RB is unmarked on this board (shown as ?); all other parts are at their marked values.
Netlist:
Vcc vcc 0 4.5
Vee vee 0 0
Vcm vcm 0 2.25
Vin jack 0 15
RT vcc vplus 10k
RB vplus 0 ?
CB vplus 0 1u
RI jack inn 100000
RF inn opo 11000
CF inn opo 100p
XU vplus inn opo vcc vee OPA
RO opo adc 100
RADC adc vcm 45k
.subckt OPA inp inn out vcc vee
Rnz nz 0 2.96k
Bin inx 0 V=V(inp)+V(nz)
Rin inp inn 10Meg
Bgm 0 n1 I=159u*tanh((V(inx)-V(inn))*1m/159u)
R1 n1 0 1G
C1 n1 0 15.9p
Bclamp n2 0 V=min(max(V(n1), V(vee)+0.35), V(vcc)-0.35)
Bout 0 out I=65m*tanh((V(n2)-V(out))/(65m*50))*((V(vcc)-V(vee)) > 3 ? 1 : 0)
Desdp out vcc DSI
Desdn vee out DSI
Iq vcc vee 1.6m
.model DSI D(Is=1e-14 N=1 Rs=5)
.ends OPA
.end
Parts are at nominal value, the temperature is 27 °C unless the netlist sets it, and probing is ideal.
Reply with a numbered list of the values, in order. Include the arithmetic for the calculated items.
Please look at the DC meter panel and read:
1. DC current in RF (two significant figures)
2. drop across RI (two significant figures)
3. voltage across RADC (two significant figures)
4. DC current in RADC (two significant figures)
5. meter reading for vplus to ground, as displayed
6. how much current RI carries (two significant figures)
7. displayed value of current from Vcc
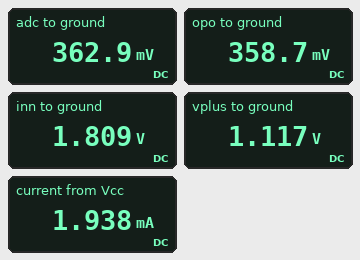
1. (1.809 V - 358.7 mV) / 11 kΩ = 130 µA
2. 15 V - 1.809 V = 13 V
3. 2.25 V - 362.9 mV = 1.9 V
4. (2.25 V - 362.9 mV) / 45 kΩ = 42 µA
5. 1.117 V
6. (15 V - 1.809 V) / 100 kΩ = 130 µA
7. 1.938 mA
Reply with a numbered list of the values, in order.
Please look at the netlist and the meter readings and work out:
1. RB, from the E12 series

1. 3.3 kΩ
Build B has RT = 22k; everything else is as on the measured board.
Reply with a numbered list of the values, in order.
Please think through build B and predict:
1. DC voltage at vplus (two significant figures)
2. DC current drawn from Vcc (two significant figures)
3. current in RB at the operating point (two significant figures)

1. 590 mV
2. 1.8 mA
3. 180 µA
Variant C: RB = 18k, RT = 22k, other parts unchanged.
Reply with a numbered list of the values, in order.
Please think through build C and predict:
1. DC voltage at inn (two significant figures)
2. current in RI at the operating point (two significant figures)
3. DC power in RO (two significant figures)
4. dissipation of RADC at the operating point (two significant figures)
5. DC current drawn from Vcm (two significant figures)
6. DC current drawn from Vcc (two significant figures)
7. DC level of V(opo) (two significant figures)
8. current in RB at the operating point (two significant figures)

1. 2.0 V
2. 130 µA
3. 130 nW
4. 60 µW
5. 37 µA
6. 1.7 mA
7. 600 mV
8. 110 µA
